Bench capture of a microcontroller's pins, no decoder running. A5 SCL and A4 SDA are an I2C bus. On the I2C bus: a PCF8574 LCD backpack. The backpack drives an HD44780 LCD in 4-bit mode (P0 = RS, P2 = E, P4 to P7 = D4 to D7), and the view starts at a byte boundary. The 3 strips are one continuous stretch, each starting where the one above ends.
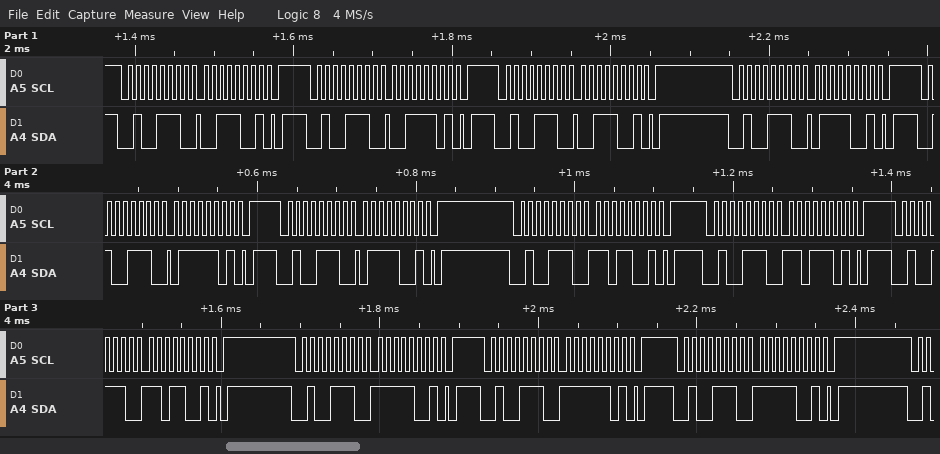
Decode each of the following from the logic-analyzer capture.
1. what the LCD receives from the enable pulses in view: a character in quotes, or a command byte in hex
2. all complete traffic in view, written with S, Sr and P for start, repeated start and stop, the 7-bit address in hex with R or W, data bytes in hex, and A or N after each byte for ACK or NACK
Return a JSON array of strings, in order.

["'7' data 0xDF", "S 27W A 39 A P S 27W A 3D A P S 27W A 39 A P S 27W A 79 A P S 27W A 7D A P S 27W A 79 A P S 27W A D9 A P S 27W A DD A P S 27W A D9 A P S 27W A F9 A P S 27W A FD A P S 27W A F9 A P"]
